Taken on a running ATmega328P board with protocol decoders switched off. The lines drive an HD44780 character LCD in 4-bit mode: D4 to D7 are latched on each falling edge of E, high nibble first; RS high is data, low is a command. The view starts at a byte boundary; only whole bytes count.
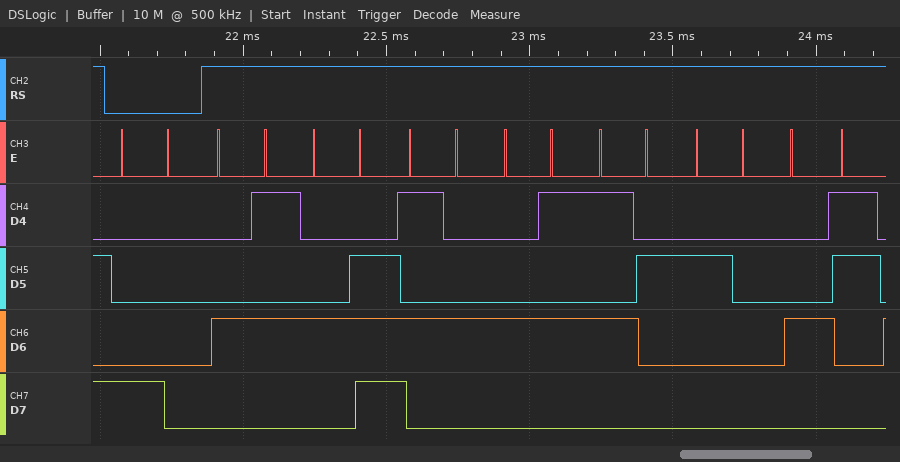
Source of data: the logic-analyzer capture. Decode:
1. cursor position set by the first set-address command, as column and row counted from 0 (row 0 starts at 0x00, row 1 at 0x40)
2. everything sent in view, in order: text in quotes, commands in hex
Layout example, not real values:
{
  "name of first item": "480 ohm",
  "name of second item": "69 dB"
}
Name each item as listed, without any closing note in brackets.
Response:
{
  "cursor position set by the first set-address command, as column and row counted from 0": "column 0, row 0",
  "everything sent in view, in order: text in quotes, commands in hex": "0x80 \"ENTER C\""
}
